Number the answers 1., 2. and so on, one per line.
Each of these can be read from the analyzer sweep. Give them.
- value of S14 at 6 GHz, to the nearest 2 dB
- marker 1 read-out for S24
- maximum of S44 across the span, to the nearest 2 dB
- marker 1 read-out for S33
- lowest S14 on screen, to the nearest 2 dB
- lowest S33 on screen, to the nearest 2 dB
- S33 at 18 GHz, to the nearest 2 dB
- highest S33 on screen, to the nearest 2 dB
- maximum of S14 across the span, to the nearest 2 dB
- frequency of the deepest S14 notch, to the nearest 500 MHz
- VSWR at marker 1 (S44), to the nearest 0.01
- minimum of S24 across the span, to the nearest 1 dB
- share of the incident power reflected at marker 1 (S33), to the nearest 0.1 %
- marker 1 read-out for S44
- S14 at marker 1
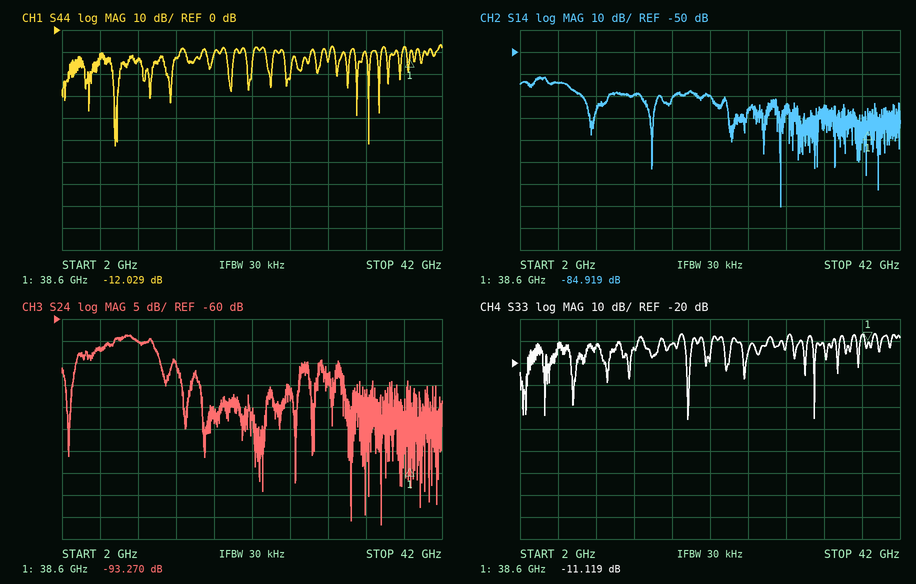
1. -64 dB
2. -93.270 dB
3. -6 dB
4. -11.119 dB
5. -120 dB
6. -46 dB
7. -12 dB
8. -6 dB
9. -62 dB
10. 29.5 GHz
11. 1.67
12. -107 dB
13. 7.7 %
14. -12.029 dB
15. -84.919 dB
